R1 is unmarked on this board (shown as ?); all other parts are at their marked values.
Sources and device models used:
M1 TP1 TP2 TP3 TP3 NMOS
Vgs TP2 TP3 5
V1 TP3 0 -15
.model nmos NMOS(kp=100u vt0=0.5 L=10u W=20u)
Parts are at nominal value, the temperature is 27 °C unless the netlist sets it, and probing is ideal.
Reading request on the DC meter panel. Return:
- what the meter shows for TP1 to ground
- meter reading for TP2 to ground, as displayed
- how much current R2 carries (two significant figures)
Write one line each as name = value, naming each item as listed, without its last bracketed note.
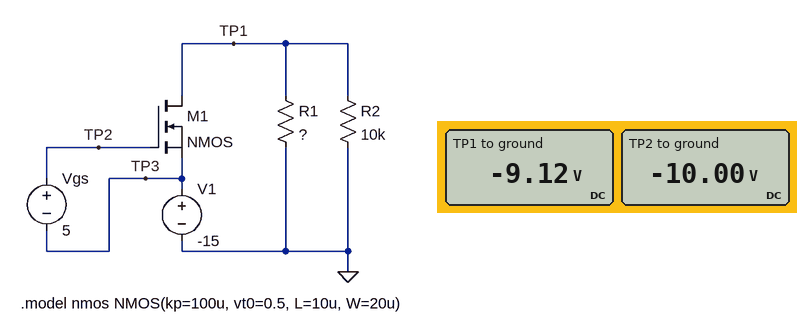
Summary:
what the meter shows for TP1 to ground = -9.12 V
meter reading for TP2 to ground, as displayed = -10.00 V
how much current R2 carries = 910 µA
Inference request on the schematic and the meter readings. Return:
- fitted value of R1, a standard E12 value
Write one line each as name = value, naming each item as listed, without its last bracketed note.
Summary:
fitted value of R1, a standard E12 value = 8.2 kΩ
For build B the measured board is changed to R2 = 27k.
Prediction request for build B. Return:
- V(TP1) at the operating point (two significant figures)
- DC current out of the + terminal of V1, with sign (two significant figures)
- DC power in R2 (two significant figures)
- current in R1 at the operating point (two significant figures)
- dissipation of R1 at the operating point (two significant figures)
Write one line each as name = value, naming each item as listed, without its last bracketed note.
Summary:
V(TP1) at the operating point = -12 V
DC current out of the + terminal of V1, with sign = -1.9 mA
DC power in R2 = 5.1 mW
current in R1 at the operating point = 1.4 mA
dissipation of R1 at the operating point = 17 mW
